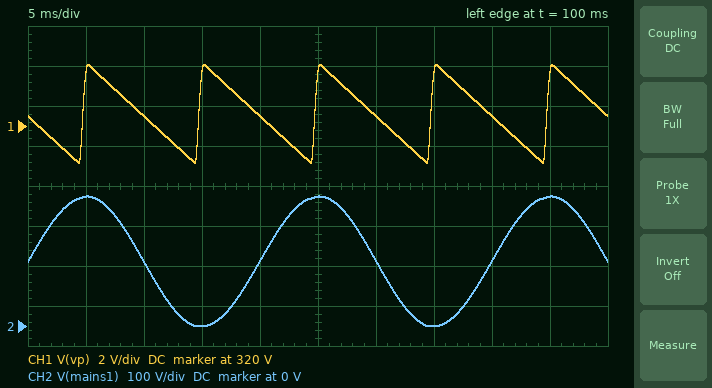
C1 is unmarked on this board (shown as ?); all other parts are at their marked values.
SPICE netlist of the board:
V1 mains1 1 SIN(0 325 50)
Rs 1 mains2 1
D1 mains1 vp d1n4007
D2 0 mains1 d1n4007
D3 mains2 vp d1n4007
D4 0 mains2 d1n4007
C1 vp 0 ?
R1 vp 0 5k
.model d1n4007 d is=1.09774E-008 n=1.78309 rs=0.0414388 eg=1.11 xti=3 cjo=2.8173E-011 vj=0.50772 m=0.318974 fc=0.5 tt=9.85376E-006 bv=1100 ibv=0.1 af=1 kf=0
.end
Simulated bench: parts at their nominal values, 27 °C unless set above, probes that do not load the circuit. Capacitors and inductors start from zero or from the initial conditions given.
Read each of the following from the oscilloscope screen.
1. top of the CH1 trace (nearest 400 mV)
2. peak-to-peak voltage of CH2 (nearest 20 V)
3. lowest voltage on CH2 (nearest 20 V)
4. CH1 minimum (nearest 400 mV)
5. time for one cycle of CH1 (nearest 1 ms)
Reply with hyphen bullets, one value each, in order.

- 323.2 V
- 320 V
- 0 V
- 318.0 V
- 10 ms
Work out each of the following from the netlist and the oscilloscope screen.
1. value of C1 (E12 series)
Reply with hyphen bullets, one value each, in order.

- 120 µF
